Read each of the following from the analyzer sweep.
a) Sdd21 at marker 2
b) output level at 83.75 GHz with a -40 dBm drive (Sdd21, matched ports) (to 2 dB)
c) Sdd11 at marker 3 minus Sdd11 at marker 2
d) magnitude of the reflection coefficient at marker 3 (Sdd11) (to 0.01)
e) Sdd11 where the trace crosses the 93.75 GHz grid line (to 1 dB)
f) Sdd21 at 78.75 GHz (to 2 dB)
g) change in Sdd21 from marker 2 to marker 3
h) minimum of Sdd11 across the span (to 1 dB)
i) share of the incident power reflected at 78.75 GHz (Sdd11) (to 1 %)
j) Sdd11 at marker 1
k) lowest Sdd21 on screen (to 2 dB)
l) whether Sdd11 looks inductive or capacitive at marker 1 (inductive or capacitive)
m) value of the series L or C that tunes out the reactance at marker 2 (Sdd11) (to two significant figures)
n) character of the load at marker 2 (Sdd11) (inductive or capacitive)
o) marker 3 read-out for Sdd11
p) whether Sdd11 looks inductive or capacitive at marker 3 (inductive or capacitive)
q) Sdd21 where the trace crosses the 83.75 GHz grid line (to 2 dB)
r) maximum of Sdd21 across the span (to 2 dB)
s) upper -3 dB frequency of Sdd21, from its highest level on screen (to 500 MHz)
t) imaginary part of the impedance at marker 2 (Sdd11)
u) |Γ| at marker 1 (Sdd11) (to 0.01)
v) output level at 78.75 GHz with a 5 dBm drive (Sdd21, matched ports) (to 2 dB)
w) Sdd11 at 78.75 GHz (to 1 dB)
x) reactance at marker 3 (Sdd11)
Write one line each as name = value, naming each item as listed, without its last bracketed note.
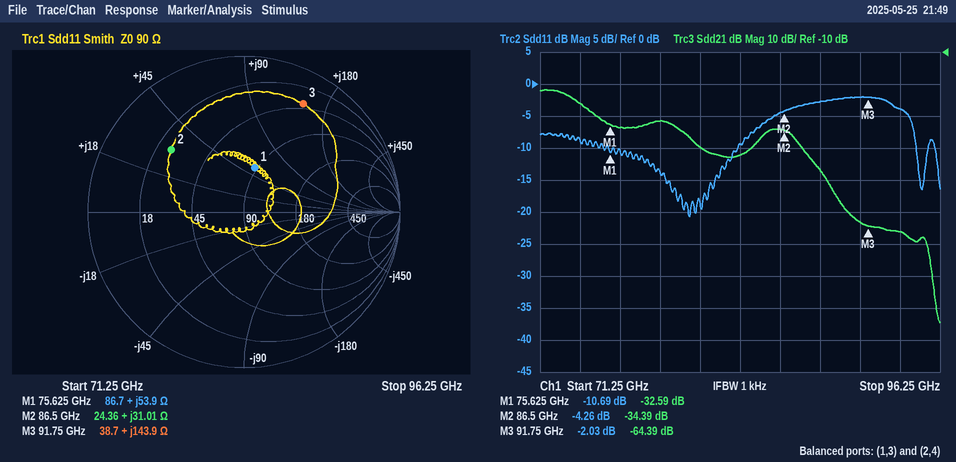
Sdd21 at marker 2 = -34.39 dB
output level at 83.75 GHz with a -40 dBm drive (Sdd21, matched ports) = -82 dBm
Sdd11 at marker 3 minus Sdd11 at marker 2 = 2.23 dB
magnitude of the reflection coefficient at marker 3 (Sdd11) = 0.79
Sdd11 where the trace crosses the 93.75 GHz grid line = -4 dB
Sdd21 at 78.75 GHz = -32 dB
change in Sdd21 from marker 2 to marker 3 = -30.00 dB
minimum of Sdd11 across the span = -21 dB
share of the incident power reflected at 78.75 GHz (Sdd11) = 4 %
Sdd11 at marker 1 = -10.69 dB
lowest Sdd21 on screen = -94 dB
whether Sdd11 looks inductive or capacitive at marker 1 = inductive
value of the series L or C that tunes out the reactance at marker 2 (Sdd11) = 59 fF
character of the load at marker 2 (Sdd11) = inductive
marker 3 read-out for Sdd11 = -2.03 dB
whether Sdd11 looks inductive or capacitive at marker 3 = inductive
Sdd21 where the trace crosses the 83.75 GHz grid line = -42 dB
maximum of Sdd21 across the span = -22 dB
upper -3 dB frequency of Sdd21, from its highest level on screen = 73.5 GHz
imaginary part of the impedance at marker 2 = +31.01 Ω
|Γ| at marker 1 (Sdd11) = 0.29
output level at 78.75 GHz with a 5 dBm drive (Sdd21, matched ports) = -26 dBm
Sdd11 at 78.75 GHz = -14 dB
reactance at marker 3 = +143.9 Ω
